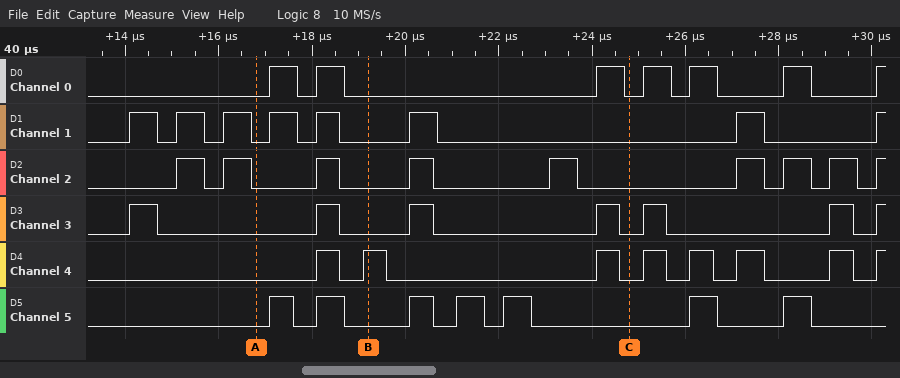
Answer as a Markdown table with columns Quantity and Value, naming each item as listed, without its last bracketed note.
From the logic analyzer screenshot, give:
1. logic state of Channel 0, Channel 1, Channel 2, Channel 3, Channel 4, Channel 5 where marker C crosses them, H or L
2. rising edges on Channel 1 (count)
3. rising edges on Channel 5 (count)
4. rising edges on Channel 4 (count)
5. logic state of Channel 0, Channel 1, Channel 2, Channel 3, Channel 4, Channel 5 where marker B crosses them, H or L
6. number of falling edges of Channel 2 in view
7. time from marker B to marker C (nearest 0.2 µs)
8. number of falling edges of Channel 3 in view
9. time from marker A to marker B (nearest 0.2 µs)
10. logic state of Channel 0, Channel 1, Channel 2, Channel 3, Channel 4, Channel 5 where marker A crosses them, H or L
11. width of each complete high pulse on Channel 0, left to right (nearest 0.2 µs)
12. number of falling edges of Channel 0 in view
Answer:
| Quantity | Value |
|---|---|
| logic state of Channel 0, Channel 1, Channel 2, Channel 3, Channel 4, Channel 5 where marker C crosses them, H or L | Channel 0=L, Channel 1=L, Channel 2=L, Channel 3=L, Channel 4=L, Channel 5=L |
| rising edges on Channel 1 | 8 |
| rising edges on Channel 5 | 7 |
| rising edges on Channel 4 | 8 |
| logic state of Channel 0, Channel 1, Channel 2, Channel 3, Channel 4, Channel 5 where marker B crosses them, H or L | Channel 0=L, Channel 1=L, Channel 2=L, Channel 3=L, Channel 4=H, Channel 5=L |
| number of falling edges of Channel 2 in view | 8 |
| time from marker B to marker C | 5.6 µs |
| number of falling edges of Channel 3 in view | 6 |
| time from marker A to marker B | 2.4 µs |
| logic state of Channel 0, Channel 1, Channel 2, Channel 3, Channel 4, Channel 5 where marker A crosses them, H or L | Channel 0=L, Channel 1=L, Channel 2=L, Channel 3=L, Channel 4=L, Channel 5=L |
| width of each complete high pulse on Channel 0, left to right | 0.6 µs, 0.6 µs, 0.6 µs, 0.6 µs, 0.6 µs, 0.6 µs |
| number of falling edges of Channel 0 in view | 6 |
